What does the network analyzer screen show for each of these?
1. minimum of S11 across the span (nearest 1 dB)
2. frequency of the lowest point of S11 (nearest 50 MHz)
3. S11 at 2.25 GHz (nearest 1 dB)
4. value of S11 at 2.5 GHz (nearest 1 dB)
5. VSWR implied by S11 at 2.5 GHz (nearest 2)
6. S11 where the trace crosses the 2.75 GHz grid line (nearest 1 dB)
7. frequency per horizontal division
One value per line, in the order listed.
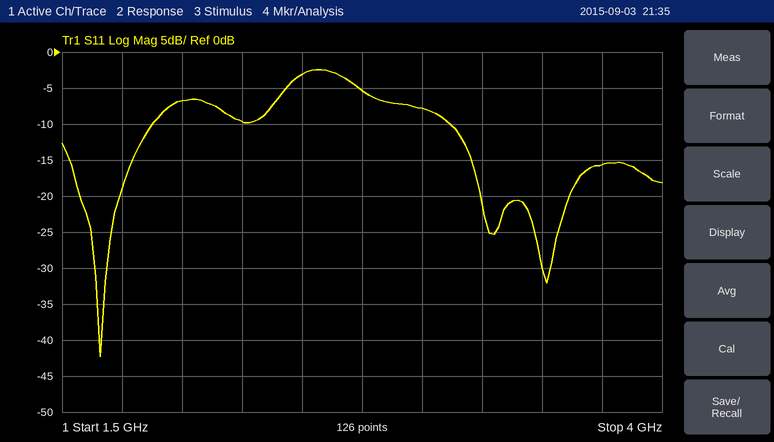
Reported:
-42 dB
1.65 GHz
-10 dB
-3 dB
6
-5 dB
250 MHz
